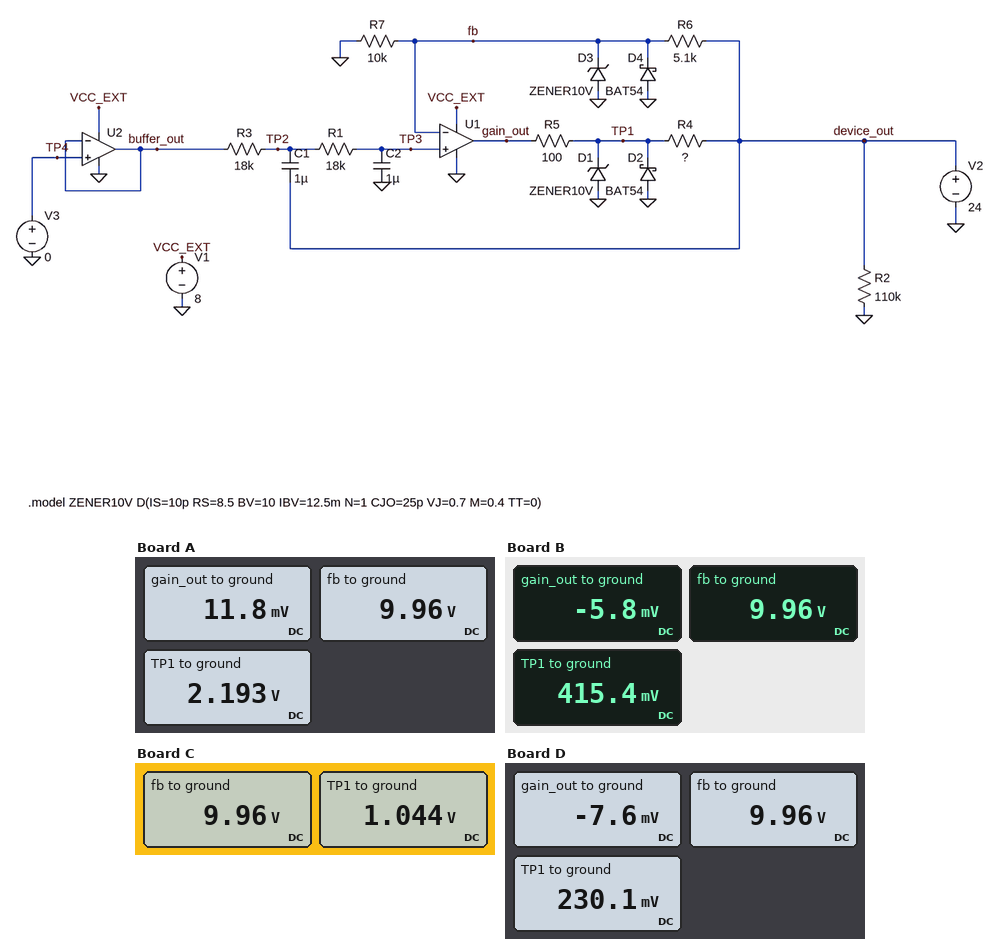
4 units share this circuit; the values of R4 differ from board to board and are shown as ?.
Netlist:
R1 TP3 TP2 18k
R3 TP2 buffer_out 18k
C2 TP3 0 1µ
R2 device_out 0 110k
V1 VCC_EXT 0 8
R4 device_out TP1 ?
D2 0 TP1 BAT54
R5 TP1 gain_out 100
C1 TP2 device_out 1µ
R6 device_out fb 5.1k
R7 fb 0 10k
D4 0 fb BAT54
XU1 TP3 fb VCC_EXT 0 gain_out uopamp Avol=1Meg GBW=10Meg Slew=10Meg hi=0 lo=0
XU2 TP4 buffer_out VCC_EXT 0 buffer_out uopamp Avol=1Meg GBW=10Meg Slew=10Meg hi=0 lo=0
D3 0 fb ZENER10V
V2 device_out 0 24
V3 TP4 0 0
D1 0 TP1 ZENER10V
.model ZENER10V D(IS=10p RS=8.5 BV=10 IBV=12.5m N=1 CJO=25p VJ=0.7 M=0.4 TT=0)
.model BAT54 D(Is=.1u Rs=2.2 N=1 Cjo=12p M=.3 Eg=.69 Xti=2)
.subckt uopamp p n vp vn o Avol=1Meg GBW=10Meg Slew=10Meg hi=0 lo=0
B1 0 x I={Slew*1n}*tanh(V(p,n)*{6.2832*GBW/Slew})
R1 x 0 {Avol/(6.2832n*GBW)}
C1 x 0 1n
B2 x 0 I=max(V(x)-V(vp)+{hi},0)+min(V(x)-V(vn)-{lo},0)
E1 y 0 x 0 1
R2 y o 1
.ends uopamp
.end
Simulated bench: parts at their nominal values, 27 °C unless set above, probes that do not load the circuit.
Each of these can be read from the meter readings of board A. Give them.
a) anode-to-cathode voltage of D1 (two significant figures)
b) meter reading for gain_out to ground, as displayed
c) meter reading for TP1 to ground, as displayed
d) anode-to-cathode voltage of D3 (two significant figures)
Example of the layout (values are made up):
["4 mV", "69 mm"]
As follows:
["-2.2 V", "11.8 mV", "2.193 V", "-10 V"]
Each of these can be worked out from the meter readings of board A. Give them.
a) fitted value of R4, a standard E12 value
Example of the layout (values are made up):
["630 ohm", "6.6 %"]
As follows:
["1 kΩ"]
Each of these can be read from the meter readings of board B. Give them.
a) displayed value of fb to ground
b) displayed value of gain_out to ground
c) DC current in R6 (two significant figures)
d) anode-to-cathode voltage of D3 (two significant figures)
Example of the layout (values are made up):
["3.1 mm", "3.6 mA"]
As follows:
["9.96 V", "-5.8 mV", "2.8 mA", "-10 V"]
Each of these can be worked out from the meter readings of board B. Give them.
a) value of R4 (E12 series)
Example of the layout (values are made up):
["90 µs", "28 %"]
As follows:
["5.6 kΩ"]
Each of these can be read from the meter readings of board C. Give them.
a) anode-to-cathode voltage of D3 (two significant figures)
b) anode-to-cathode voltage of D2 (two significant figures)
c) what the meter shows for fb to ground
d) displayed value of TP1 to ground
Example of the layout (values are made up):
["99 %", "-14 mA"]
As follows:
["-10 V", "-1.0 V", "9.96 V", "1.044 V"]
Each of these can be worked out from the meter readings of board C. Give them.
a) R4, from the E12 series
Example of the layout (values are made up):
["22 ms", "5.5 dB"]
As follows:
["2.2 kΩ"]
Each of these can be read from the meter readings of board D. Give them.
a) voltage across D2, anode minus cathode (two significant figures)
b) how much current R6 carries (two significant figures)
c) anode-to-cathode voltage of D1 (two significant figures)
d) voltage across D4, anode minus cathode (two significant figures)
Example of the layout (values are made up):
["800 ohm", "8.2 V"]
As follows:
["-230 mV", "2.8 mA", "-230 mV", "-10 V"]
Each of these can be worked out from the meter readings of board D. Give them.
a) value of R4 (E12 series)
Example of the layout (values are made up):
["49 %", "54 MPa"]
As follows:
["10 kΩ"]
